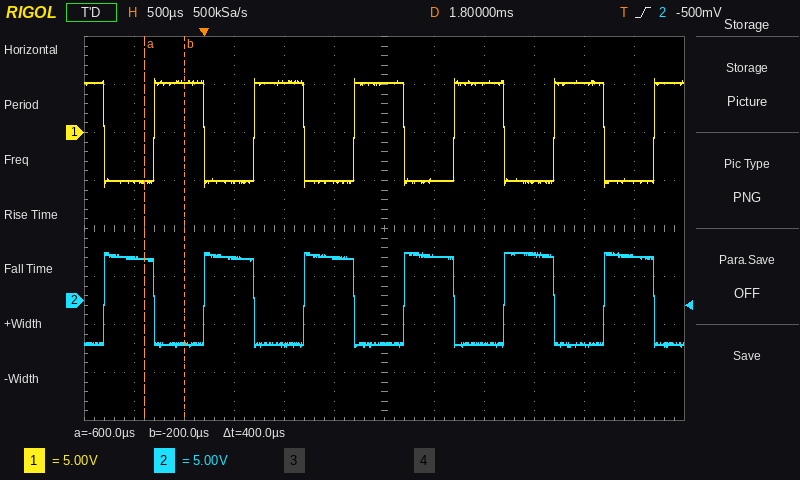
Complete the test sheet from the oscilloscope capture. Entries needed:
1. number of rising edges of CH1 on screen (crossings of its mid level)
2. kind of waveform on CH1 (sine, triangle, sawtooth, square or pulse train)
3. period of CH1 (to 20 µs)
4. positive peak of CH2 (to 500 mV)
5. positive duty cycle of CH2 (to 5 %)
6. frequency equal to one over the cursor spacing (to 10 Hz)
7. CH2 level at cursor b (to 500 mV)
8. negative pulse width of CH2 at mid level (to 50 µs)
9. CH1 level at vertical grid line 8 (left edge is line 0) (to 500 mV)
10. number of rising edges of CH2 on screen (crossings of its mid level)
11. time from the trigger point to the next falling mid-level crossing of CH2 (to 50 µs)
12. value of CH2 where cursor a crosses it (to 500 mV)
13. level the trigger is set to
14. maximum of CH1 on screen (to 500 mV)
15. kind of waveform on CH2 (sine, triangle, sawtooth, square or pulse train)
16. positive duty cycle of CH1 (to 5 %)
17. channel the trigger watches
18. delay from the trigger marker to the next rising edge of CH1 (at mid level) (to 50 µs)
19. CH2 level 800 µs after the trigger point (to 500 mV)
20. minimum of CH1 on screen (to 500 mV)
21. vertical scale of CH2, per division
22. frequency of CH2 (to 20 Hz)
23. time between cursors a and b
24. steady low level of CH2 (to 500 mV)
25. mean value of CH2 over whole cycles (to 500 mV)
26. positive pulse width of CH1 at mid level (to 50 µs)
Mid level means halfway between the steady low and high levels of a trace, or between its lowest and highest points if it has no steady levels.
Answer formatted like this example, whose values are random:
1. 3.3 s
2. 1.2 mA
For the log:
1. 6
2. square
3. 1.00 ms
4. 5.0 V
5. 50 %
6. 2.50 kHz
7. -4.5 V
8. 500 µs
9. 5.0 V
10. 6
11. 500 µs
12. 4.5 V
13. -500 mV
14. 5.5 V
15. square
16. 50 %
17. CH2
18. 500 µs
19. -4.5 V
20. -5.5 V
21. 5 V
22. 1.00 kHz
23. 400 µs
24. -4.5 V
25. 0.0 V
26. 500 µs
